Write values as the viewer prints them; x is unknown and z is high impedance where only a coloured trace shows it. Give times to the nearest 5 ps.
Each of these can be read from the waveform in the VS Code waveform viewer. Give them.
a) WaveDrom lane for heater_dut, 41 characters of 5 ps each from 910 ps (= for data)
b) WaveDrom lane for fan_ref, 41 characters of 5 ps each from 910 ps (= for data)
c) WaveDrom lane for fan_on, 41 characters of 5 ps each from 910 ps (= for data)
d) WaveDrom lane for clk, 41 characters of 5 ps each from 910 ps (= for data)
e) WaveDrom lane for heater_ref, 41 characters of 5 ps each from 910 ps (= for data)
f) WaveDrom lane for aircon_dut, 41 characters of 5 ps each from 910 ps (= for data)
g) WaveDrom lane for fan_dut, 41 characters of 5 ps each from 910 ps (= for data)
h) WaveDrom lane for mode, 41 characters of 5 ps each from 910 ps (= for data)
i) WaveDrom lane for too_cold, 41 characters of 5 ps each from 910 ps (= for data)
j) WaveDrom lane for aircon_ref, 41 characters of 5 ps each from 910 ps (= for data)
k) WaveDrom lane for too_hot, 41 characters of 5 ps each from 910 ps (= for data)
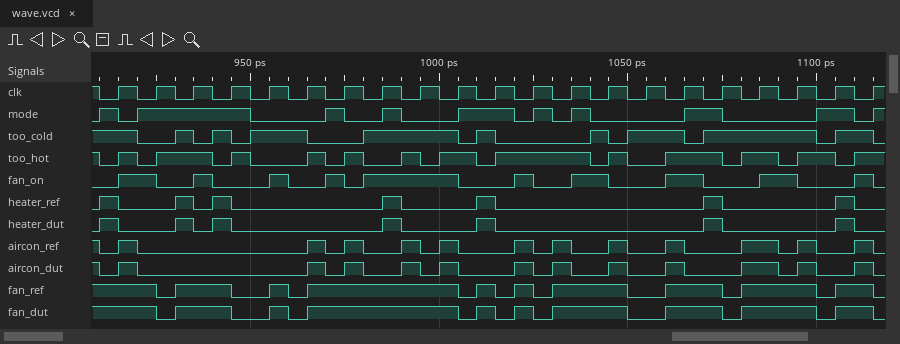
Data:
{name: 'heater_dut', wave: '10..1010.......10...10..........10.....10'}
{name: 'fan_ref', wave: '1..01..0.101.......010101...0.1..01...01.'}
{name: 'fan_on', wave: '01.0.10..10.101....0..10.1.0..1.0..1.0..1'}
{name: 'clk', wave: '01010101010101010101010101010101010101010'}
{name: 'heater_ref', wave: '10..1010.......10...10..........10.....10'}
{name: 'aircon_dut', wave: '010........1010.1010..1010.10.10..1.010.1'}
{name: 'fan_dut', wave: '1..01..0.101.......010101...0.1..01...01.'}
{name: 'mode', wave: '101.....0...10.10..1..01010....1.0....1.0'}
{name: 'too_cold', wave: '1.0.10101..0..1....010....101..01.....01.'}
{name: 'aircon_ref', wave: '010........1010.1010..1010.10.10..1.010.1'}
{name: 'too_hot', wave: '0101..010..1010.101.01....010.1..01.01.01'}
